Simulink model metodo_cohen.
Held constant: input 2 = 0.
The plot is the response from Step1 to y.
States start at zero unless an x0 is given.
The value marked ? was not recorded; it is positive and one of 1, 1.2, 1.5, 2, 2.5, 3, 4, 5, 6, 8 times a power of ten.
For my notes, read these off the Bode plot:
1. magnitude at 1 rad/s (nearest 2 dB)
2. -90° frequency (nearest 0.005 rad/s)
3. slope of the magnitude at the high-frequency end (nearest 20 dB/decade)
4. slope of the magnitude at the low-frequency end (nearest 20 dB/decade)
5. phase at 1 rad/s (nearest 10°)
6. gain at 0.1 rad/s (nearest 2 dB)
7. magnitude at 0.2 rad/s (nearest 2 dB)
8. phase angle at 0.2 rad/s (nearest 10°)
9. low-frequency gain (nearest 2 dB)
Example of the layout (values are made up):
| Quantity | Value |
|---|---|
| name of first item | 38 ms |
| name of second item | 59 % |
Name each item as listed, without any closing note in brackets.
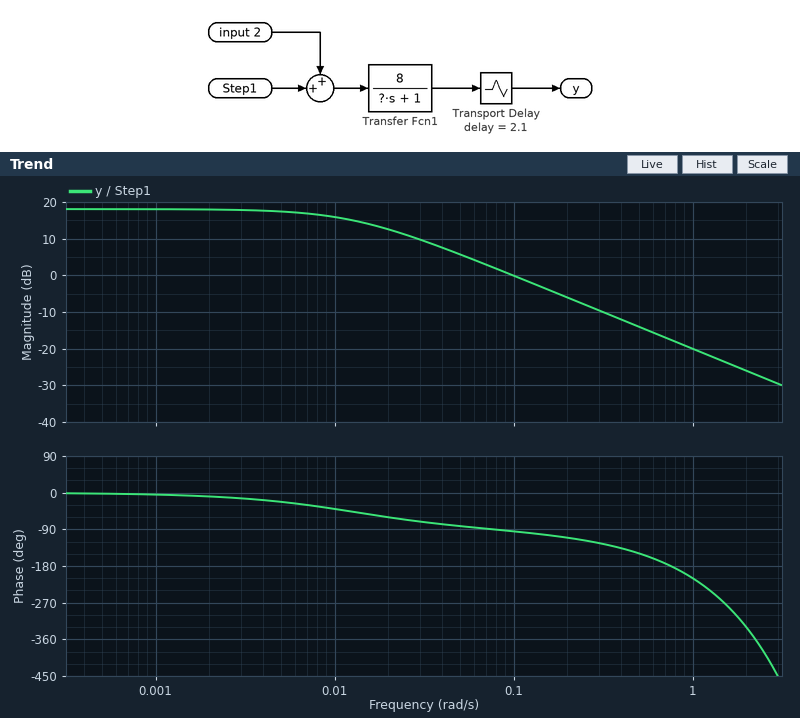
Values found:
| Quantity | Value |
|---|---|
| magnitude at 1 rad/s | -20 dB |
| -90° frequency | 0.075 rad/s |
| slope of the magnitude at the high-frequency end | -20 dB/decade |
| slope of the magnitude at the low-frequency end | 0 dB/decade |
| phase at 1 rad/s | -210° |
| gain at 0.1 rad/s | 0 dB |
| magnitude at 0.2 rad/s | -6 dB |
| phase angle at 0.2 rad/s | -110° |
| low-frequency gain | 18 dB |
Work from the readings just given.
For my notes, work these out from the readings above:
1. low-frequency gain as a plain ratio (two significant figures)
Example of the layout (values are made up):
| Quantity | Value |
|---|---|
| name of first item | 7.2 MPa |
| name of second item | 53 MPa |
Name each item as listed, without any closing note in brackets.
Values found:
| Quantity | Value |
|---|---|
| low-frequency gain as a plain ratio | 7.9 |
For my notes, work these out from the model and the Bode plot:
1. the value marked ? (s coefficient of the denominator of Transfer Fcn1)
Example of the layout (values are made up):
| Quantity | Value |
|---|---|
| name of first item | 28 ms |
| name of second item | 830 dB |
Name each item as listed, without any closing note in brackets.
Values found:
| Quantity | Value |
|---|---|
| the value marked ? | 80 |
